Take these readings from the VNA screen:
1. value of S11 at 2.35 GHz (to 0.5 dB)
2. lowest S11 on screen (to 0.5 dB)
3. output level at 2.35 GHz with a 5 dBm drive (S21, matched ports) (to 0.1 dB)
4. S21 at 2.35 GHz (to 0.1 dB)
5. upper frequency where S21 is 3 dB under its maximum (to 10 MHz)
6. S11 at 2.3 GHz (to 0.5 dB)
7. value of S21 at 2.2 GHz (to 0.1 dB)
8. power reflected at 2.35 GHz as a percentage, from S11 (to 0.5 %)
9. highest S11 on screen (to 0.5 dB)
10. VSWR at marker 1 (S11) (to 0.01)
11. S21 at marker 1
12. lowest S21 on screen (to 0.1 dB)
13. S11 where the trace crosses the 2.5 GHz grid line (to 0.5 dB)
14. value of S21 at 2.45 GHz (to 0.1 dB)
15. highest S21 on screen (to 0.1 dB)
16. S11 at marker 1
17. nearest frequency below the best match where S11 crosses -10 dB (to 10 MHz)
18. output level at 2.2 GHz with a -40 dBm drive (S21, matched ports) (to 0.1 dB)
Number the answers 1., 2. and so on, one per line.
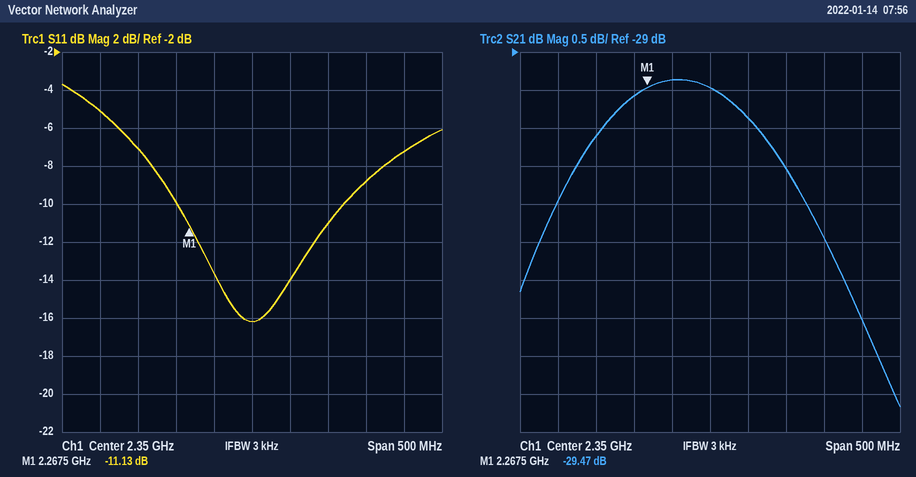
1. -16.0 dB
2. -16.0 dB
3. -24.5 dBm
4. -29.5 dB
5. 2.54 GHz
6. -13.5 dB
7. -30.1 dB
8. 2.5 %
9. -3.5 dB
10. 1.77
11. -29.47 dB
12. -33.7 dB
13. -9.0 dB
14. -30.5 dB
15. -29.4 dB
16. -11.13 dB
17. 2.25 GHz
18. -70.1 dBm
